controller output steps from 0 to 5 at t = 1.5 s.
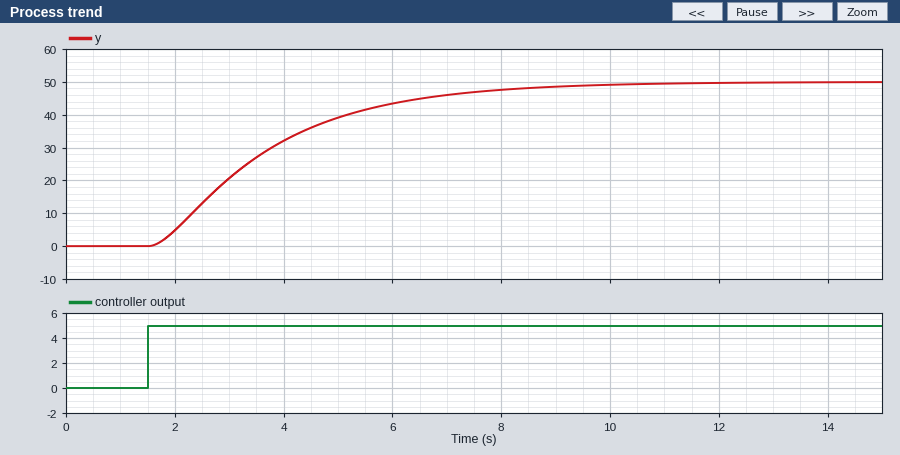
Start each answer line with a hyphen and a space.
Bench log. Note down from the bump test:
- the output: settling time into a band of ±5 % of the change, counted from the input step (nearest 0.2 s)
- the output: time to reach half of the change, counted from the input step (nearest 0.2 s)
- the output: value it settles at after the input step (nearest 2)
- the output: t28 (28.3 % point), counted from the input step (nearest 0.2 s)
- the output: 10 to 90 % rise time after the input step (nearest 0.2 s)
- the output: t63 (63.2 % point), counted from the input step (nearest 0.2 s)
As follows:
- 6.4 s
- 1.8 s
- 50
- 1.0 s
- 4.6 s
- 2.4 s
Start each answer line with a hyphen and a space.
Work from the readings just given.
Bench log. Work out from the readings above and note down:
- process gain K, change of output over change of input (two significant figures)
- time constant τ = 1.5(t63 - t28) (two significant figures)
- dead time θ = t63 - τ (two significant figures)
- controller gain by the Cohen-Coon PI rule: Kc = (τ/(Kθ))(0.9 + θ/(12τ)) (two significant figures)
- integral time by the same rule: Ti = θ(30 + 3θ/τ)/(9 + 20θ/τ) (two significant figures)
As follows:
- 10
- 2.1 s
- 0.30 s
- 0.64
- 0.77 s
